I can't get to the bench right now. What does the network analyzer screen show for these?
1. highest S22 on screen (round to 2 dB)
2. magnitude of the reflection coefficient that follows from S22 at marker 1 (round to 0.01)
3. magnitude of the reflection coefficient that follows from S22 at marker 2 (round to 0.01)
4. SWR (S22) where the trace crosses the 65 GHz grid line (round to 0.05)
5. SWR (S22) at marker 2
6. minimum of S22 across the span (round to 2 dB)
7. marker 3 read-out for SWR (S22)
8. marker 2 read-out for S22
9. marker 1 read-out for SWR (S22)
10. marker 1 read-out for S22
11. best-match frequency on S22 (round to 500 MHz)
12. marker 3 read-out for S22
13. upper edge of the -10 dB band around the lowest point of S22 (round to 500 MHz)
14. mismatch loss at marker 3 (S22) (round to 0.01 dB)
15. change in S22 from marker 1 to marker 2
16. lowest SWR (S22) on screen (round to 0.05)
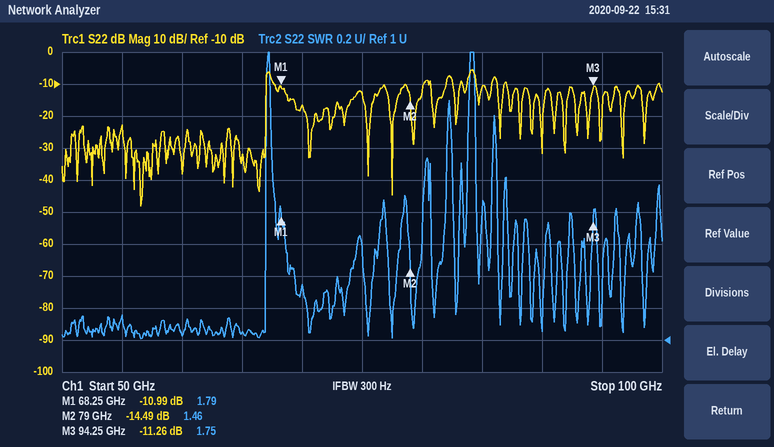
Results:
-6 dB
0.28
0.19
1.05
1.46
-48 dB
1.75
-14.49 dB
1.79
-10.99 dB
56.5 GHz
-11.26 dB
67.0 GHz
0.34 dB
-3.50 dB
1.00
